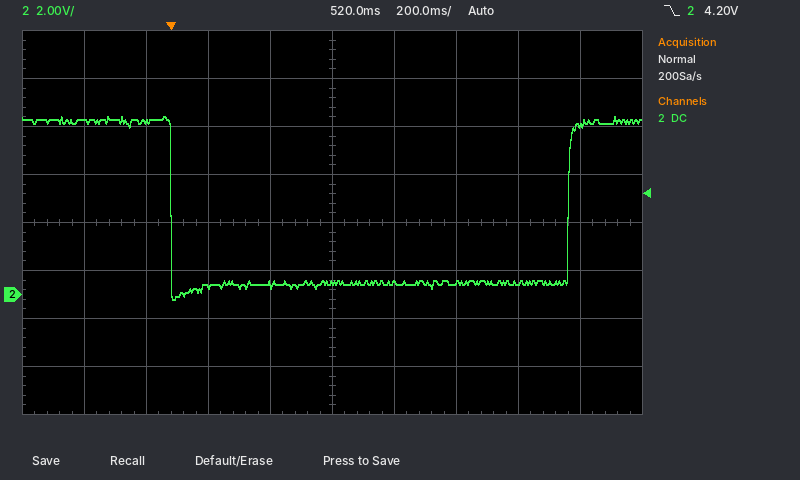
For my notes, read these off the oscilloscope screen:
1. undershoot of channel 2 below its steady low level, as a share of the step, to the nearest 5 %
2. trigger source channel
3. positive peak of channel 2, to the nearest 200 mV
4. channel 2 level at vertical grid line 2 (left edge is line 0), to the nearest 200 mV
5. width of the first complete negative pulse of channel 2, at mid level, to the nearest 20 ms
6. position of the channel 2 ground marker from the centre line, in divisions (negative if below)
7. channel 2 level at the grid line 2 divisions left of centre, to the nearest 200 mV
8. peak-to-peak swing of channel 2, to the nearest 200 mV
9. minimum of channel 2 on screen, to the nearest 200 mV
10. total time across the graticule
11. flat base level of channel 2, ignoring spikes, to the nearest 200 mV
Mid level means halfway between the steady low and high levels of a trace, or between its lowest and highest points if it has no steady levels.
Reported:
10 %
channel 2
7.4 V
7.2 V
1.28 s
-1.5 div
400 mV
7.6 V
-200 mV
2 s
400 mV
